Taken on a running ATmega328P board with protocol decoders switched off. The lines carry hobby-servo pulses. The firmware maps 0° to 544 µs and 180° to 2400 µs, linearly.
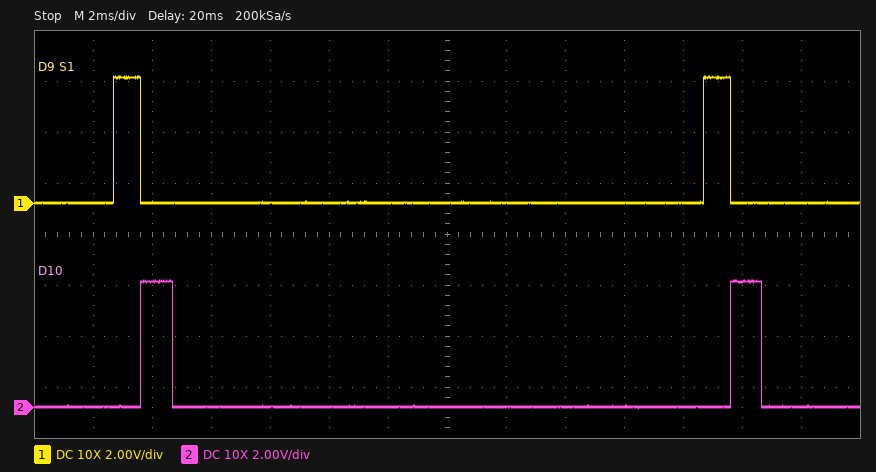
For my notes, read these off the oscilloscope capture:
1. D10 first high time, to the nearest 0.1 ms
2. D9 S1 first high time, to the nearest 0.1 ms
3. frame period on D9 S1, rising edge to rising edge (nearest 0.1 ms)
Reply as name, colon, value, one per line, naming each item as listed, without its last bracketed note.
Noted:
D10 first high time, to the nearest 0.1 ms: 1.1 ms
D9 S1 first high time, to the nearest 0.1 ms: 0.9 ms
frame period on D9 S1, rising edge to rising edge: 20.0 ms
